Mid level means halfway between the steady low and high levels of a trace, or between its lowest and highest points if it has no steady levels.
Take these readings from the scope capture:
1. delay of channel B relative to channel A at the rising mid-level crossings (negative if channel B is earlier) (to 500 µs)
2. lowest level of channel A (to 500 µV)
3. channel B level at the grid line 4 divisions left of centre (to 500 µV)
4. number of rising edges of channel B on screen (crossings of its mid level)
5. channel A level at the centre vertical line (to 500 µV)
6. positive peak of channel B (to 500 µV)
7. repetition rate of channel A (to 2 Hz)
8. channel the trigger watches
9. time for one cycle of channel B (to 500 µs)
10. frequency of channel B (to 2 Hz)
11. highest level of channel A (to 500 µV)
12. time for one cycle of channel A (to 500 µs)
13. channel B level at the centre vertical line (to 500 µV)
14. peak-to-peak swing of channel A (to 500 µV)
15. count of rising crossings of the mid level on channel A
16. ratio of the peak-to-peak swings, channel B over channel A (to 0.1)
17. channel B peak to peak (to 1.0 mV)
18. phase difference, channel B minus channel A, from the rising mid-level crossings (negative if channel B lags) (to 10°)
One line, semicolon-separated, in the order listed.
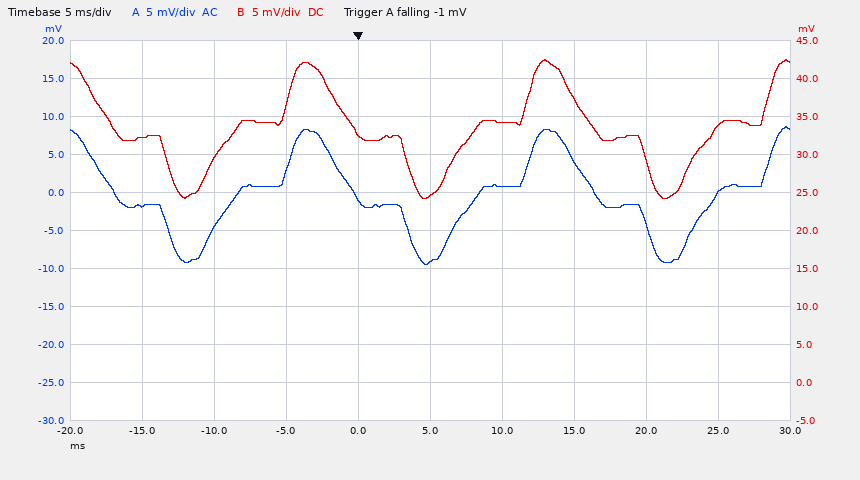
0.0 ms; -9.5 mV; 32.0 mV; 3; -9.0 mV; 42.5 mV; 60 Hz; channel A; 16.5 ms; 60 Hz; 8.5 mV; 16.5 ms; 24.5 mV; 18.0 mV; 3; 1.0; 18.0 mV; 0°
